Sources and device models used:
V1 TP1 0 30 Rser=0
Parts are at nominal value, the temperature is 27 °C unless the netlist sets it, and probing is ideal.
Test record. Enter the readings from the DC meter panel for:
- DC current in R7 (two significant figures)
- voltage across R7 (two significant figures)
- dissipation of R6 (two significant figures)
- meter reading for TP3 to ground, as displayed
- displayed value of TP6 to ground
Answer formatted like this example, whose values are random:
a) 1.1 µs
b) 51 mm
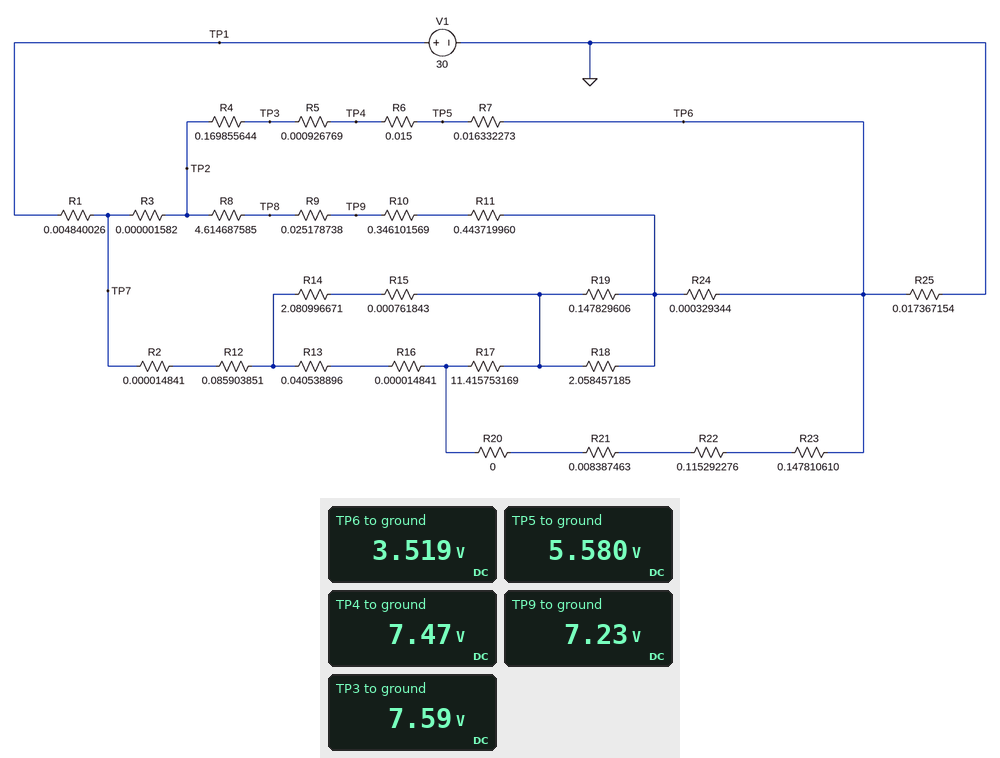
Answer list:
a) 130 A
b) 2.1 V
c) 240 W
d) 7.59 V
e) 3.519 V
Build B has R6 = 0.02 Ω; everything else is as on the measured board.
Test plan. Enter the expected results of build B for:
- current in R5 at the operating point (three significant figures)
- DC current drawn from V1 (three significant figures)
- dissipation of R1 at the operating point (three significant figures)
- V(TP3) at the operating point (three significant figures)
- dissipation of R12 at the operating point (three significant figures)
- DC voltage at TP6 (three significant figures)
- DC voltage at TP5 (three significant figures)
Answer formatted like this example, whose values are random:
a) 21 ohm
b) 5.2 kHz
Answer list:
a) 123 A
b) 200 A
c) 194 W
d) 8.07 V
e) 444 W
f) 3.47 V
g) 5.49 V
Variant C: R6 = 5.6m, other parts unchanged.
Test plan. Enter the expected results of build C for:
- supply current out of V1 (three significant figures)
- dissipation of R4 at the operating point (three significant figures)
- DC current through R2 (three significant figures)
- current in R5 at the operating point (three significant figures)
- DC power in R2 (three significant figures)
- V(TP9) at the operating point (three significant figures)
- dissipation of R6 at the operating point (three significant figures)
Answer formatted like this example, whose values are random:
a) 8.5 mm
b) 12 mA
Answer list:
a) 208 A
b) 2.95 kW
c) 71.4 A
d) 132 A
e) 75.7 mW
f) 7.31 V
g) 97.2 W
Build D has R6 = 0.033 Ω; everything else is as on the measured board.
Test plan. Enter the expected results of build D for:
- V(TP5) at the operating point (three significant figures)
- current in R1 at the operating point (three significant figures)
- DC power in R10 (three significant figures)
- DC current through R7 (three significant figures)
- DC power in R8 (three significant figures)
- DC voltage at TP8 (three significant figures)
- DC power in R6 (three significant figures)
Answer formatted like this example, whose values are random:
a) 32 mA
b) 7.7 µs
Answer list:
a) 5.27 V
b) 194 A
c) 7.75 W
d) 117 A
e) 103 W
f) 7.23 V
g) 450 W
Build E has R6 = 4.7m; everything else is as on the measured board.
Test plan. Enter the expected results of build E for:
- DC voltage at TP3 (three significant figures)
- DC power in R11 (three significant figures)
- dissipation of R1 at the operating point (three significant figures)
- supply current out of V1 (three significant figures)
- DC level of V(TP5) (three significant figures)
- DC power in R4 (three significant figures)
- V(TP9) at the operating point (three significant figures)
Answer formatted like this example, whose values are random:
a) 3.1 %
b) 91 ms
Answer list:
a) 6.52 V
b) 9.69 W
c) 210 W
d) 208 A
e) 5.78 V
f) 2.97 kW
g) 7.31 V
